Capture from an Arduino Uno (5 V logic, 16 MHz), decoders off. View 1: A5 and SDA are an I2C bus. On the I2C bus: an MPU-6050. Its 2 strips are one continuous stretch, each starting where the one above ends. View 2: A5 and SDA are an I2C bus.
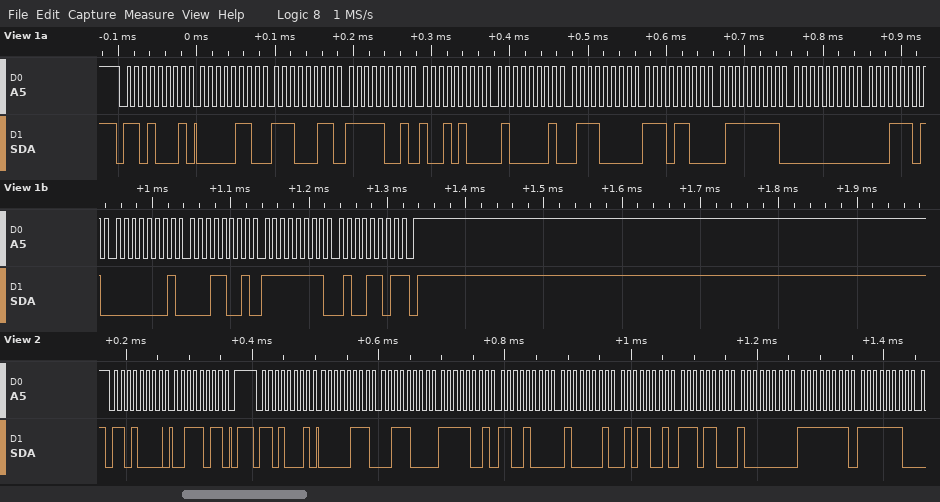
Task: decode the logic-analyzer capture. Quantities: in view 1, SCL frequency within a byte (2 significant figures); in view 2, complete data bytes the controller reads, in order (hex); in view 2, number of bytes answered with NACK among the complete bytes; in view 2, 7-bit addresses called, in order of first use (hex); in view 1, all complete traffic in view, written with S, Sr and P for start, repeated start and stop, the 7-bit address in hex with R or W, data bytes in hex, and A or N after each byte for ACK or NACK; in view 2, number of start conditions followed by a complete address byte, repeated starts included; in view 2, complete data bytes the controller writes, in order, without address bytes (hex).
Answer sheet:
100 kHz
07 38 F9 C8 41 59 EC 80 FF FE
0
0x68
S 68R A 06 A E3 A F9 A 94 A 41 A 70 A EC A 7F A 00 A 1D A 01 A 19 A FF A 4D N P
2
3B
